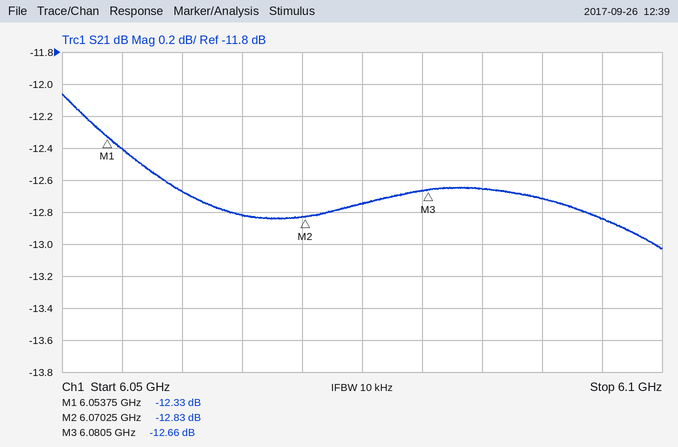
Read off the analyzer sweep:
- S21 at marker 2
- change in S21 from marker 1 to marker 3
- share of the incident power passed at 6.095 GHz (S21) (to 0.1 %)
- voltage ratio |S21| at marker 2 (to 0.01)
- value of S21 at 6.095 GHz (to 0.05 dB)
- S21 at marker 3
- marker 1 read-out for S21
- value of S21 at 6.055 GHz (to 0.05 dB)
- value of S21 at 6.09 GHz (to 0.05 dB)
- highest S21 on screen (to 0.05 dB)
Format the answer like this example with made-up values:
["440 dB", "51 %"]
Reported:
["-12.83 dB", "-0.33 dB", "5.2 %", "0.23", "-12.85 dB", "-12.66 dB", "-12.33 dB", "-12.40 dB", "-12.70 dB", "-12.05 dB"]
